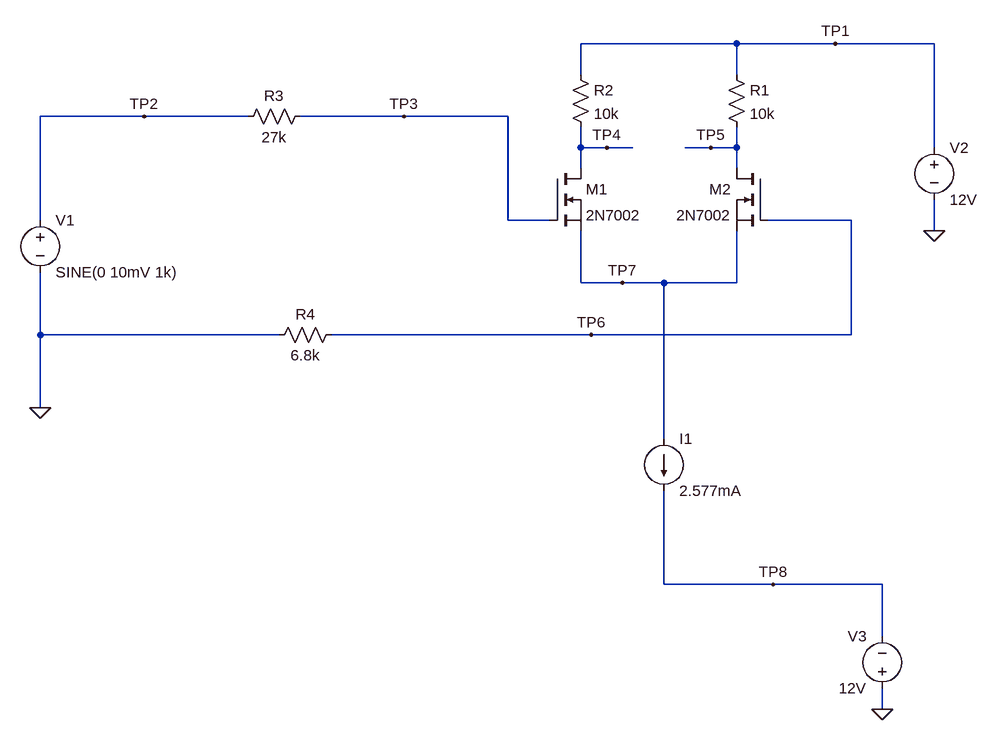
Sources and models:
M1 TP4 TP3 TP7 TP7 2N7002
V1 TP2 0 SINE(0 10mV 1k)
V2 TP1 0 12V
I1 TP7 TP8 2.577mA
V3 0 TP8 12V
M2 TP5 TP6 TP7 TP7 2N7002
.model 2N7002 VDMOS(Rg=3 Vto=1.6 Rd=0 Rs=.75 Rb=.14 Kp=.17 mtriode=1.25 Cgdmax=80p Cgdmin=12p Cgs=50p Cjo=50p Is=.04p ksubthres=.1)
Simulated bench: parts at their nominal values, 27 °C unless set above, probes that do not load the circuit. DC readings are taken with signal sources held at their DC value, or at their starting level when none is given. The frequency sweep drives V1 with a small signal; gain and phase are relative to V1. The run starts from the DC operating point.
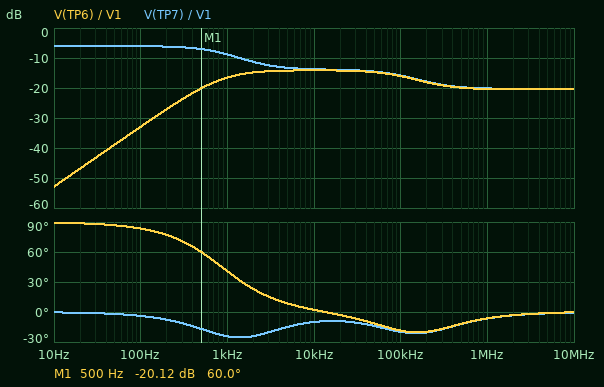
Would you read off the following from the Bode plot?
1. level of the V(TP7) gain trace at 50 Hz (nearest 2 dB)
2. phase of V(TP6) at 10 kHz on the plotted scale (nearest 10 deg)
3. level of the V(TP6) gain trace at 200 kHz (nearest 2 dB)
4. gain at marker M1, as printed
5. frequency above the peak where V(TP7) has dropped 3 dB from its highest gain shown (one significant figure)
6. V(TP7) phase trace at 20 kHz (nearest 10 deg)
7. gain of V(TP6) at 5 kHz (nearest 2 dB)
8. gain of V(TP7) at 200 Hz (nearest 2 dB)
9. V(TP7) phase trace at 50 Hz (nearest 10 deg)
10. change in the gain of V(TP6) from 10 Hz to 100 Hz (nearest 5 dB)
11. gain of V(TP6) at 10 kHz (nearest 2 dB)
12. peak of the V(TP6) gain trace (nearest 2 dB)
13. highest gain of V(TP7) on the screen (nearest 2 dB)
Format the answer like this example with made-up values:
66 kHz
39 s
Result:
-6 dB
0 deg
-18 dB
-20.12 dB
1 kHz
-10 deg
-14 dB
-6 dB
0 deg
20 dB
-14 dB
-14 dB
-6 dB
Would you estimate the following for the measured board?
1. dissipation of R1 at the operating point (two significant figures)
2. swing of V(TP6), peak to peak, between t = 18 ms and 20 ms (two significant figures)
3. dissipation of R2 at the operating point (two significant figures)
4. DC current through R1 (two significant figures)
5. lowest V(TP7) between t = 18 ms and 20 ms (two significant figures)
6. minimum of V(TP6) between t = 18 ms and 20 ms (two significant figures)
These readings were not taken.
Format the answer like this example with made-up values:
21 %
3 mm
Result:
17 mW
3.0 mV
17 mW
1.3 mA
-1.7 V
-1.5 mV
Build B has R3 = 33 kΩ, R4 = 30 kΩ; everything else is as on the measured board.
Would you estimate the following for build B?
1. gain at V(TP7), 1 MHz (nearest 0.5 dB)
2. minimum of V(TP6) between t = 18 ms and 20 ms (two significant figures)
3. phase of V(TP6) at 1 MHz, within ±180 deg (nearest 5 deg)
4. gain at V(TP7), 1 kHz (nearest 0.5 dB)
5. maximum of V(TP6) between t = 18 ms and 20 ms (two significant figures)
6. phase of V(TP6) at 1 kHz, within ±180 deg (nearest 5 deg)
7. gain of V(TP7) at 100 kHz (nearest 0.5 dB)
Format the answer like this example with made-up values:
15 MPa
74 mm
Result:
-18.5 dB
-4.3 mV
-10 deg
-6.5 dB
4.3 mV
25 deg
-12.0 dB
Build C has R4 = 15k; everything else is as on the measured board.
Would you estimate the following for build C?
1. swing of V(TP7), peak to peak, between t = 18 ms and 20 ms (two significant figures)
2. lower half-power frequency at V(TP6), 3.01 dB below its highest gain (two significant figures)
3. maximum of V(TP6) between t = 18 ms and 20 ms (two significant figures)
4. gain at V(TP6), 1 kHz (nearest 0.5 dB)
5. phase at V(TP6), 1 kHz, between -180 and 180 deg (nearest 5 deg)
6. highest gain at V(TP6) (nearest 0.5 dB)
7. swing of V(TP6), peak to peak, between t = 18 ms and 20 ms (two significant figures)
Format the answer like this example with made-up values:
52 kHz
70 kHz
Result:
8.2 mV
690 Hz
2.9 mV
-11.0 dB
35 deg
-9.0 dB
5.8 mV
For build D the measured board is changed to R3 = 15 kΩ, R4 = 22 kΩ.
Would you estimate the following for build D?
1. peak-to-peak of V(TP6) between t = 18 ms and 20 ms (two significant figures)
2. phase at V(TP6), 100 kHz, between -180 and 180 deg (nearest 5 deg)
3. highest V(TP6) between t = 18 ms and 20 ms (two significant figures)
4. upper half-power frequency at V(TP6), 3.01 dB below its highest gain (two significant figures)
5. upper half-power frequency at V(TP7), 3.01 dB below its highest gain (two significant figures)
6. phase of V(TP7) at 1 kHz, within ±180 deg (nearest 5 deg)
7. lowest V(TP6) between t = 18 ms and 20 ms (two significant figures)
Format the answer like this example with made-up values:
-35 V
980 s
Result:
9.2 mV
-25 deg
4.6 mV
94 kHz
93 kHz
5 deg
-4.6 mV
